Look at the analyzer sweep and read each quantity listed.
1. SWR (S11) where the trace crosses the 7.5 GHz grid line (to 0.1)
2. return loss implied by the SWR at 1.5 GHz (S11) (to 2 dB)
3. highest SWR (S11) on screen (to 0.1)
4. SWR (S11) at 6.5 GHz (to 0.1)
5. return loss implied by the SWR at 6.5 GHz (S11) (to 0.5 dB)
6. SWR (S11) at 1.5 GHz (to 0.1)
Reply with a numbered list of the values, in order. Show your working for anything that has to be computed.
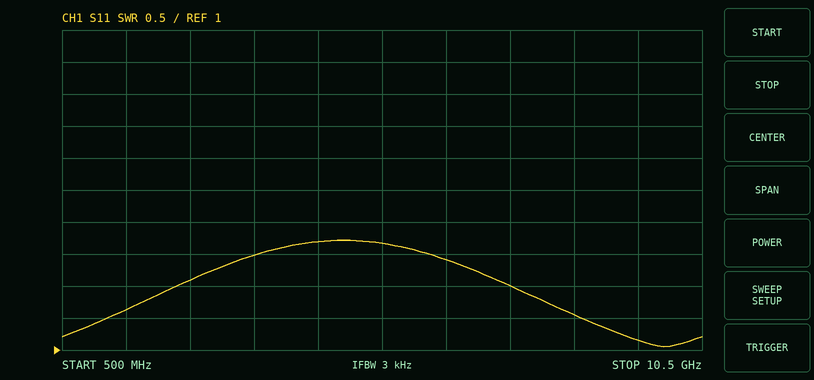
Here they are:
1. 2.0
2. −20 log10((1.6 − 1)/(1.6 + 1)) ≈ 12.7 dB, so 12 dB to the nearest 2 dB
3. 2.7
4. 2.4
5. −20 log10((2.4 − 1)/(2.4 + 1)) ≈ 7.71 dB, so 7.5 dB to the nearest 0.5 dB
6. 1.6
